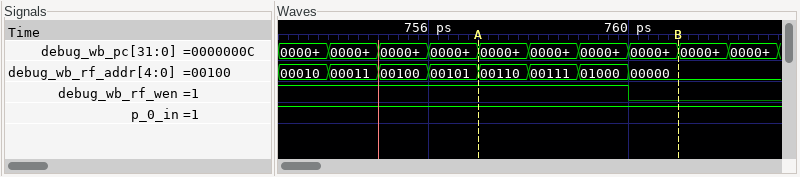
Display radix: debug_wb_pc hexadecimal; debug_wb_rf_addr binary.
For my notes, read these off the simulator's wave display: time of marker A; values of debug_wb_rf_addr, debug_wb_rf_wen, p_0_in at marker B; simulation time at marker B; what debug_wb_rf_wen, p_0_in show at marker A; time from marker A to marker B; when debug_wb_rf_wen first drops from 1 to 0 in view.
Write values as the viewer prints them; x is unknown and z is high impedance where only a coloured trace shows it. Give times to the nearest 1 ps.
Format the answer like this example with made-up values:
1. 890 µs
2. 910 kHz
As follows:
1. 757 ps
2. debug_wb_rf_addr=00000, debug_wb_rf_wen=0, p_0_in=1
3. 761 ps
4. debug_wb_rf_wen=1, p_0_in=1
5. 4 ps
6. 760 ps
